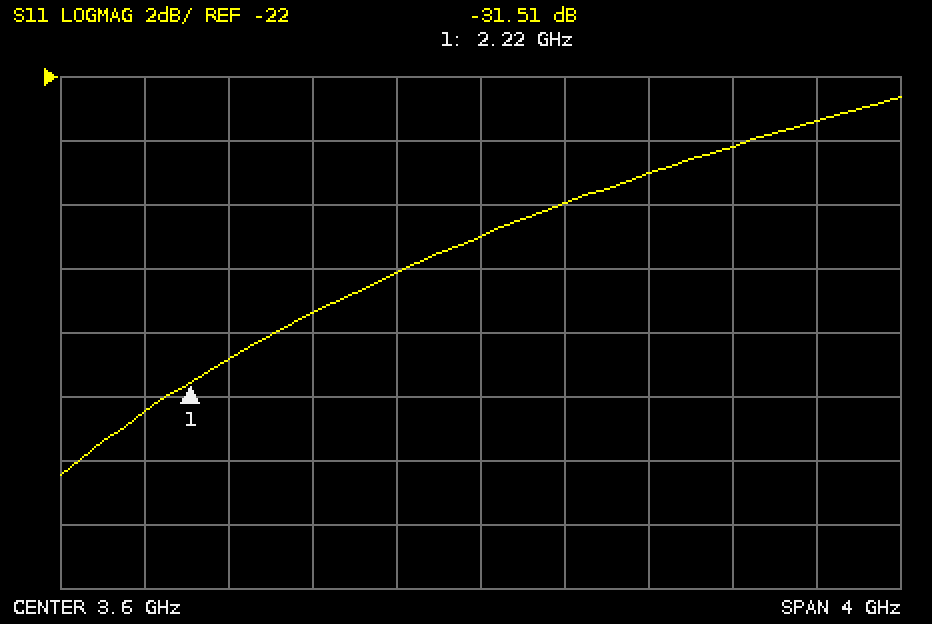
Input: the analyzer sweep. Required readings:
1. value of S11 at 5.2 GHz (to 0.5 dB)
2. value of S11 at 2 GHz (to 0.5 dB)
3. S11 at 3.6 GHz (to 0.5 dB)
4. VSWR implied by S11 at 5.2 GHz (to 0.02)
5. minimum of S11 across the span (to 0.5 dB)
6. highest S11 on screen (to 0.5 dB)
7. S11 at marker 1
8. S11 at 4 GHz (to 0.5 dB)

-23.5 dB
-32.5 dB
-27.0 dB
1.14
-34.5 dB
-22.5 dB
-31.51 dB
-26.0 dB
